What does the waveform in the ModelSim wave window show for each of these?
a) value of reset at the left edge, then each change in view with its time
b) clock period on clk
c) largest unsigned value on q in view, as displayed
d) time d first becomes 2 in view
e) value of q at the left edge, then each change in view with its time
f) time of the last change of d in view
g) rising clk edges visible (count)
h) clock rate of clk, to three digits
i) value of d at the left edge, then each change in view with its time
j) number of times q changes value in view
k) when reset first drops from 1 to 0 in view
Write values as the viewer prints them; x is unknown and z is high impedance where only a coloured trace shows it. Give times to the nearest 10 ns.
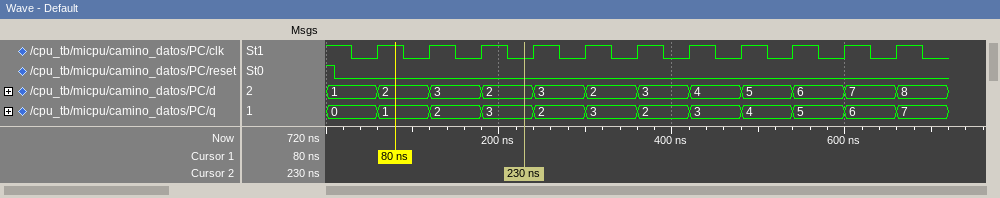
1, 0 at 10 ns
60 ns
7
60 ns
0, 1 at 60 ns, 2 at 120 ns, 3 at 180 ns, 2 at 240 ns, 3 at 300 ns, 2 at 360 ns, 3 at 420 ns, 4 at 480 ns, 5 at 540 ns, 6 at 600 ns, 7 at 660 ns
660 ns
11
16.7 MHz
1, 2 at 60 ns, 3 at 120 ns, 2 at 180 ns, 3 at 240 ns, 2 at 300 ns, 3 at 360 ns, 4 at 420 ns, 5 at 480 ns, 6 at 540 ns, 7 at 600 ns, 8 at 660 ns
11
10 ns
